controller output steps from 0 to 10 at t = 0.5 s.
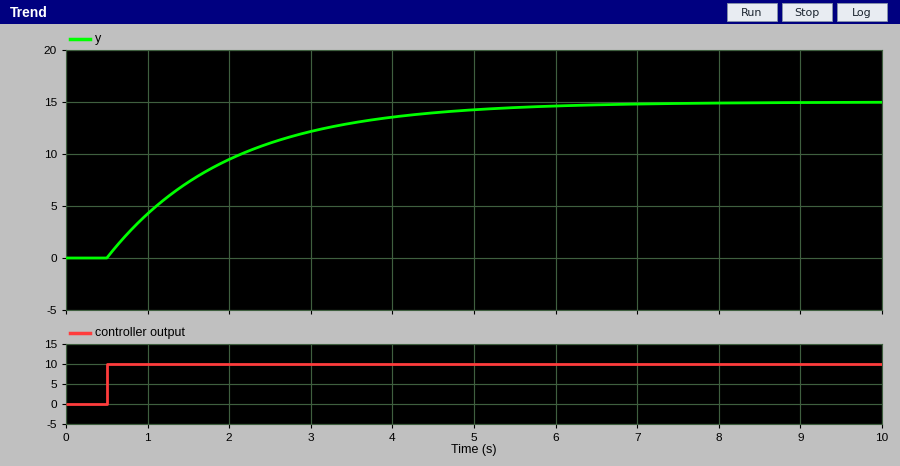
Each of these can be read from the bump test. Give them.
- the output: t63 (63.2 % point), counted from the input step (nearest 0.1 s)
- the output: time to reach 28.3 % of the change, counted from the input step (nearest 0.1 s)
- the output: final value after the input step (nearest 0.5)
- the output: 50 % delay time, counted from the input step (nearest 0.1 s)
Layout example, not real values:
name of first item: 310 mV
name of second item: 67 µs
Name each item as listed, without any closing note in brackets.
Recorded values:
the output: t63 (63.2 % point), counted from the input step: 1.5 s
the output: time to reach 28.3 % of the change, counted from the input step: 0.5 s
the output: final value after the input step: 15.0
the output: 50 % delay time, counted from the input step: 1.0 s
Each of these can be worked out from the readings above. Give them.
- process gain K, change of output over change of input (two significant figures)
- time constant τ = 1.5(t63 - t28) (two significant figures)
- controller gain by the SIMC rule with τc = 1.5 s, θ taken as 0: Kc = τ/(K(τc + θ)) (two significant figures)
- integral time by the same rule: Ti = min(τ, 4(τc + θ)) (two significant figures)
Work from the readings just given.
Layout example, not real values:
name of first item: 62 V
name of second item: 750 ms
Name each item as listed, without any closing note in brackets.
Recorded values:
process gain K, change of output over change of input: 1.5
time constant τ = 1.5(t63 - t28): 1.5 s
controller gain by the SIMC rule with τc = 1.5 s, θ taken as 0: Kc = τ/(K(τc + θ)): 0.67
integral time by the same rule: Ti = min(τ, 4(τc + θ)): 1.5 s
